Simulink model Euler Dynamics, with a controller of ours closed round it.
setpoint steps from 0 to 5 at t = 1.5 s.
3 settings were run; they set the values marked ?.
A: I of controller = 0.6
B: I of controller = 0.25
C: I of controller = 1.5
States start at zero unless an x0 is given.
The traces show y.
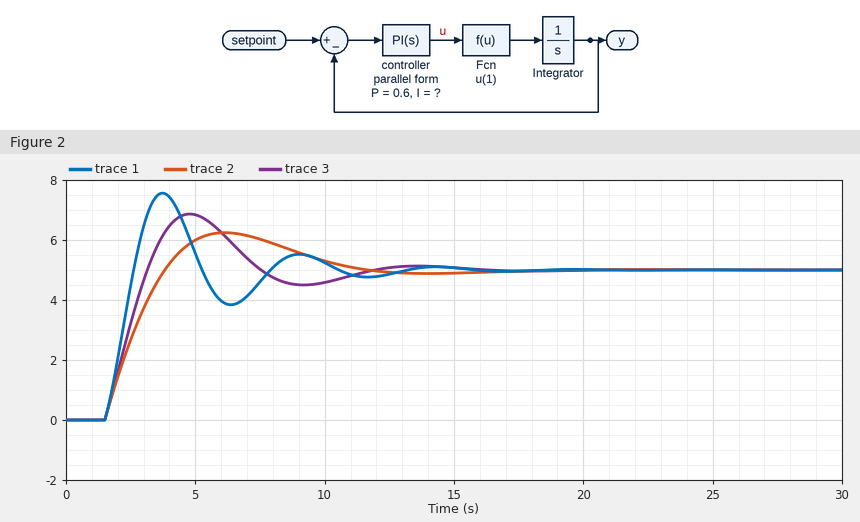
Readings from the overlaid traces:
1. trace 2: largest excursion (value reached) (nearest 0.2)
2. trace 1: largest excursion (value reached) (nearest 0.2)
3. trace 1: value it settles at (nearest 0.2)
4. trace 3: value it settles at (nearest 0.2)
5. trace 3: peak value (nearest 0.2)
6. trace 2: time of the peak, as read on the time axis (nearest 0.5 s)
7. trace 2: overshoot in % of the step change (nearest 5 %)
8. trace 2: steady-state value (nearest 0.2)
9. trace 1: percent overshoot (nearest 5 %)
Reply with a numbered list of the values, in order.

1. 6.2
2. 7.6
3. 5.0
4. 5.0
5. 6.8
6. 6.0 s
7. 25 %
8. 5.0
9. 50 %
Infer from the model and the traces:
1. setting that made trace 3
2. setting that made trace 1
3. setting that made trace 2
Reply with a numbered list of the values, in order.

1. A
2. C
3. B
